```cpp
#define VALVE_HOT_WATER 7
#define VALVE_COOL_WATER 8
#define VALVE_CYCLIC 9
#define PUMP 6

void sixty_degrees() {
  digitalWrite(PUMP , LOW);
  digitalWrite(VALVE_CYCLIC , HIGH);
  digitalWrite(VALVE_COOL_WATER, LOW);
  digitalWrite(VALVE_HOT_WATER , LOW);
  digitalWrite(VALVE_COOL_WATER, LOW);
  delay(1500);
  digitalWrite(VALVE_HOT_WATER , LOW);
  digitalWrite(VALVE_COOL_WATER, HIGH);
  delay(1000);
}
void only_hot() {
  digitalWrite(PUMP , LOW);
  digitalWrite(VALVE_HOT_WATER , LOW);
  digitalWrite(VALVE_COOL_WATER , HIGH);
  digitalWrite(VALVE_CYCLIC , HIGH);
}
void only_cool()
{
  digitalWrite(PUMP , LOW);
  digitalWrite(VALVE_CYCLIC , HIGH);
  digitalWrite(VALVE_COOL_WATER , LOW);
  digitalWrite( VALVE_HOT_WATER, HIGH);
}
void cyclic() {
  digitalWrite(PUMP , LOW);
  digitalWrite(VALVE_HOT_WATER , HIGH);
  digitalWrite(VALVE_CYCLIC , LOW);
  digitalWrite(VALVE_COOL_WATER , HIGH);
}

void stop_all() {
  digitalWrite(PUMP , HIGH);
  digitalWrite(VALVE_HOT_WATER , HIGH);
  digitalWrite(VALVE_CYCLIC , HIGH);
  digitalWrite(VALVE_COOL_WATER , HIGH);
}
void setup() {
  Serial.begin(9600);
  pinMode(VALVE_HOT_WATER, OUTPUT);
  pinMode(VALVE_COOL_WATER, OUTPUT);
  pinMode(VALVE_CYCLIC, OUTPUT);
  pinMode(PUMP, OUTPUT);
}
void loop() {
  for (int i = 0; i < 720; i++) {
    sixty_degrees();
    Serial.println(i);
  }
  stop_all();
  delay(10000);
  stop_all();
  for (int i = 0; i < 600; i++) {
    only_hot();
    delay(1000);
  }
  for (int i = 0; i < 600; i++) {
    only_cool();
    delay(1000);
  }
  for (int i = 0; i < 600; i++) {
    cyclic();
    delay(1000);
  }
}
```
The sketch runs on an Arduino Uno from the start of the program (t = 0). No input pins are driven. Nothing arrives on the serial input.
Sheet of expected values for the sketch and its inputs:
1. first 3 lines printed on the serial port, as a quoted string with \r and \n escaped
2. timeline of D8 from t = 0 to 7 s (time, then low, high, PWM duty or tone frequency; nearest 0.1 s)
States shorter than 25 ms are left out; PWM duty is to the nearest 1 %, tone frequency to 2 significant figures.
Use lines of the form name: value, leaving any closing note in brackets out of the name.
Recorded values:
first 3 lines printed on the serial port, as a quoted string with \r and \n escaped: "0\r\n1\r\n2\r\n"
timeline of D8 from t = 0 to 7 s: 0 s low; 1.5 s high; 2.5 s low; 4 s high; 5 s low; 6.5 s high
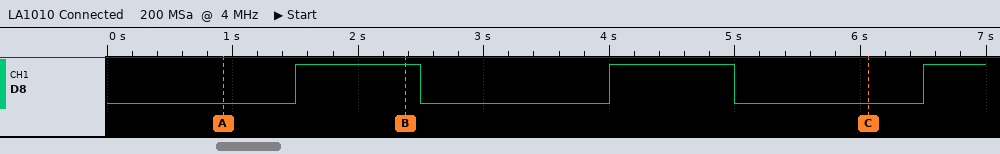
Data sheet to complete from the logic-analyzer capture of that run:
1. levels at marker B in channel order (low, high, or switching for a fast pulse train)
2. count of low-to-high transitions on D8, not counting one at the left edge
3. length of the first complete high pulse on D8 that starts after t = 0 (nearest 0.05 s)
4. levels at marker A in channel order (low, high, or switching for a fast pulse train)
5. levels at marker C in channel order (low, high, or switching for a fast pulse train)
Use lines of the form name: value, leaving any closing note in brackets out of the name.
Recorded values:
levels at marker B in channel order: D8 high
count of low-to-high transitions on D8, not counting one at the left edge: 3
length of the first complete high pulse on D8 that starts after t = 0: 1.00 s
levels at marker A in channel order: D8 low
levels at marker C in channel order: D8 low
